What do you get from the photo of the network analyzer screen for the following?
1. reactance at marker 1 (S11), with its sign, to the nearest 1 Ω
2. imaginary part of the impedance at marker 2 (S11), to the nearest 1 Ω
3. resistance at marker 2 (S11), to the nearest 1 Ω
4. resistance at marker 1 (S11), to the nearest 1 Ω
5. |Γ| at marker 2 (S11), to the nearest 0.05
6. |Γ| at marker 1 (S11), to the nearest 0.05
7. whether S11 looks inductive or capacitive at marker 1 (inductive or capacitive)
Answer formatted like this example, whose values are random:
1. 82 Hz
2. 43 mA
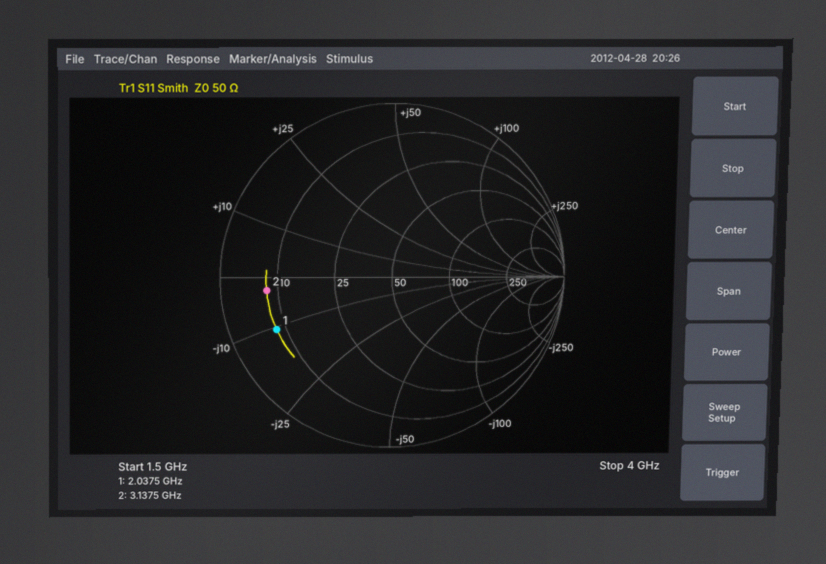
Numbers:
1. -11 Ω
2. -3 Ω
3. 8 Ω
4. 8 Ω
5. 0.75
6. 0.75
7. capacitive
